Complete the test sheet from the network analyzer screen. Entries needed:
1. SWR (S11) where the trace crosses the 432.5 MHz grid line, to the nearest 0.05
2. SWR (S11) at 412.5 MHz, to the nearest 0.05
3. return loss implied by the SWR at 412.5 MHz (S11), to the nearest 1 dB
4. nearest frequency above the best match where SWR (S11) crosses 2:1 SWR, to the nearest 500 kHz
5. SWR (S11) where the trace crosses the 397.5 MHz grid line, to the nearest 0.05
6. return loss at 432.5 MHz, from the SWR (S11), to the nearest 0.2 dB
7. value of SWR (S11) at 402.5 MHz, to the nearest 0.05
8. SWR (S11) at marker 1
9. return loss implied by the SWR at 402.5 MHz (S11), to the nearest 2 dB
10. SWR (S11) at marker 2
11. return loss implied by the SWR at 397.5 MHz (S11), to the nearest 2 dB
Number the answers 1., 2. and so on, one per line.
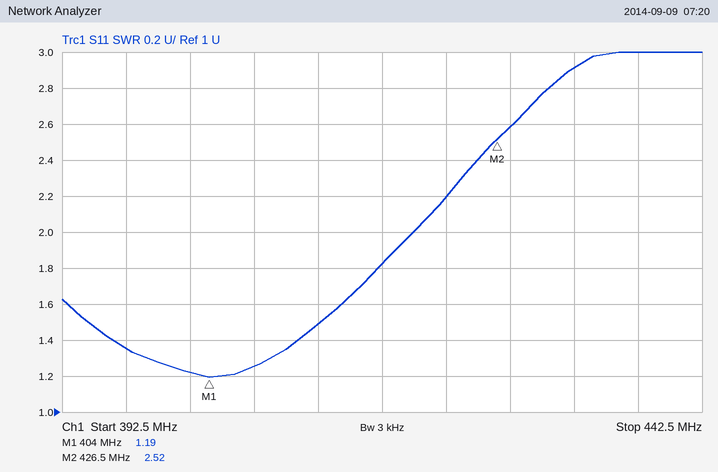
1. 2.90
2. 1.50
3. 14 dB
4. 420.0 MHz
5. 1.35
6. 6.2 dB
7. 1.20
8. 1.19
9. 20 dB
10. 2.52
11. 16 dB
